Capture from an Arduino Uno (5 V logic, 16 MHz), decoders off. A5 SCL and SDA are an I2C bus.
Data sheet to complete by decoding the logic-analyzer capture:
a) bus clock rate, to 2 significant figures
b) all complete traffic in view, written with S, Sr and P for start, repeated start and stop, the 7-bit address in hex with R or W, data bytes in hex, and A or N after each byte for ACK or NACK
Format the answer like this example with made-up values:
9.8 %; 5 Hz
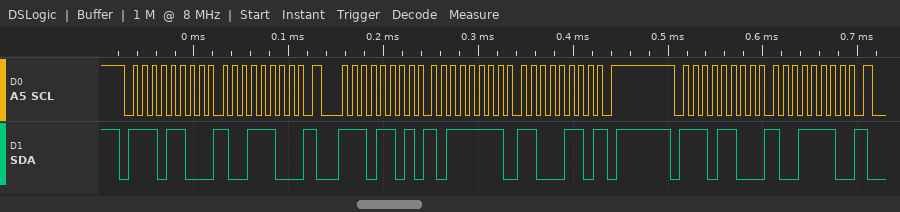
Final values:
100 kHz; S 76W A 9C A Sr 76R A BF A C6 N P S 76W A 9E A
